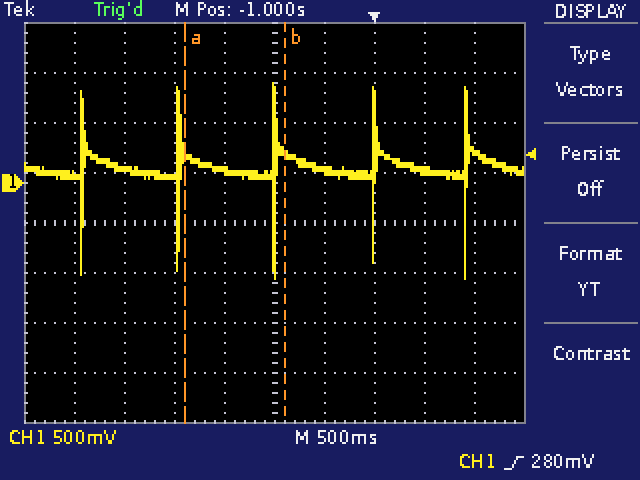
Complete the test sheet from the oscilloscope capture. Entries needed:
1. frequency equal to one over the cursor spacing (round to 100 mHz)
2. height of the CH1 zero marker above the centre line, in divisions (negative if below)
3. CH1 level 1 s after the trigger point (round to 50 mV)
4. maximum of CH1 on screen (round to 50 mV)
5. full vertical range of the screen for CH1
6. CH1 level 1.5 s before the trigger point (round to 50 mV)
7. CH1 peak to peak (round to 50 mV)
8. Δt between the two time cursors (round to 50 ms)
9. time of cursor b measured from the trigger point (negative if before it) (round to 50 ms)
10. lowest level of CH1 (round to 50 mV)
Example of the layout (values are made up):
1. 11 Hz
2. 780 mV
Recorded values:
1. 1.0 Hz
2. +0.8 div
3. 300 mV
4. 1.00 V
5. 4 V
6. 100 mV
7. 1.95 V
8. 1.00 s
9. -900 ms
10. -950 mV
